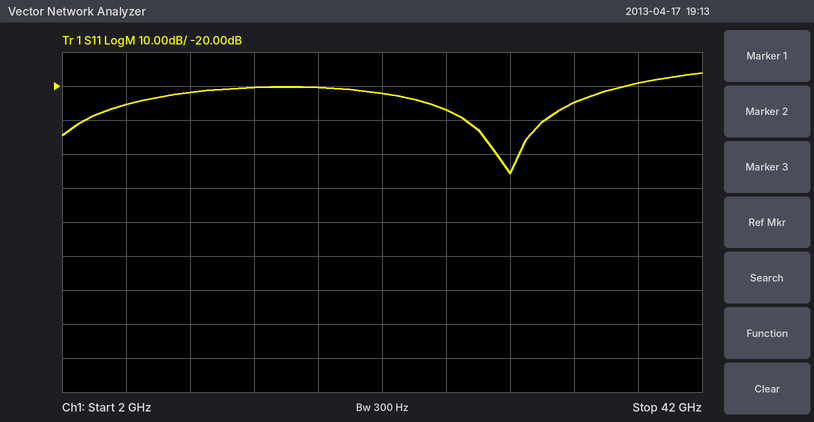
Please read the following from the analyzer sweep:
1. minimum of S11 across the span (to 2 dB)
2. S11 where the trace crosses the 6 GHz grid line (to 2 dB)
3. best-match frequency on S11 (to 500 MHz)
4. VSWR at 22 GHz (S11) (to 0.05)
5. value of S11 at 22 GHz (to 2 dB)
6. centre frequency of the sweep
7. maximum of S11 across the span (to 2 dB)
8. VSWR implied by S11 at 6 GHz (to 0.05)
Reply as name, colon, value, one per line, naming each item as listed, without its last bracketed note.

minimum of S11 across the span: -46 dB
S11 where the trace crosses the 6 GHz grid line: -26 dB
best-match frequency on S11: 30.0 GHz
VSWR at 22 GHz (S11): 1.15
value of S11 at 22 GHz: -22 dB
centre frequency of the sweep: 22 GHz
maximum of S11 across the span: -16 dB
VSWR implied by S11 at 6 GHz: 1.10
